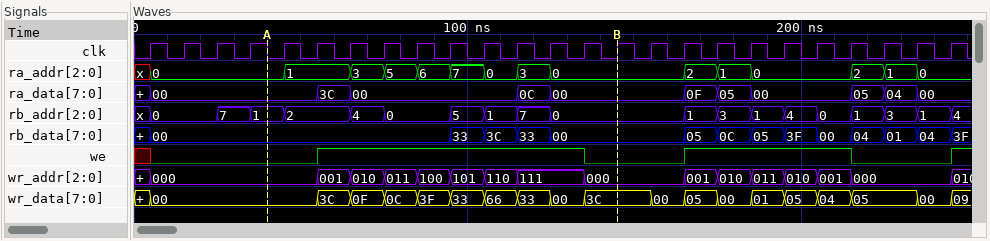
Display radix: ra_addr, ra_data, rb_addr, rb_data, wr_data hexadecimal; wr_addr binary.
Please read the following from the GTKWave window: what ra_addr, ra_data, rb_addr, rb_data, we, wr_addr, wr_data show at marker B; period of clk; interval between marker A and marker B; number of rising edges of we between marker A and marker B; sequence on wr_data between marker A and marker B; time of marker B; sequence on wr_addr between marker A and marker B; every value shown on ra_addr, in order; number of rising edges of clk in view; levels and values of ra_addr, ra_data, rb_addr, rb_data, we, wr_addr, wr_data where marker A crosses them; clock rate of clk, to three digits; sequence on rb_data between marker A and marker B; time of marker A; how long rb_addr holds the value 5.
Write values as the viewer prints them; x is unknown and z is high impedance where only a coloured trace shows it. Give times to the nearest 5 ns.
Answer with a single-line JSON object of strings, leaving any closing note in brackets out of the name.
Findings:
{"what ra_addr, ra_data, rb_addr, rb_data, we, wr_addr, wr_data show at marker B": "ra_addr=0, ra_data=00, rb_addr=0, rb_data=00, we=0, wr_addr=000, wr_data=3C", "period of clk": "10 ns", "interval between marker A and marker B": "105 ns", "number of rising edges of we between marker A and marker B": "1", "sequence on wr_data between marker A and marker B": "00, 3C, 0F, 0C, 3F, 33, 66, 33, 00, 3C", "time of marker B": "145 ns", "sequence on wr_addr between marker A and marker B": "000, 001, 010, 011, 100, 101, 110, 111, 000", "every value shown on ra_addr, in order": "x, 0, 1, 3, 5, 6, 7, 0, 3, 0, 2, 1, 0, 2, 1, 0", "number of rising edges of clk in view": "25", "levels and values of ra_addr, ra_data, rb_addr, rb_data, we, wr_addr, wr_data where marker A crosses them": "ra_addr=0, ra_data=00, rb_addr=1, rb_data=00, we=0, wr_addr=000, wr_data=00", "clock rate of clk, to three digits": "100 MHz", "sequence on rb_data between marker A and marker B": "00, 33, 3C, 33, 00", "time of marker A": "40 ns", "how long rb_addr holds the value 5": "10 ns"}
